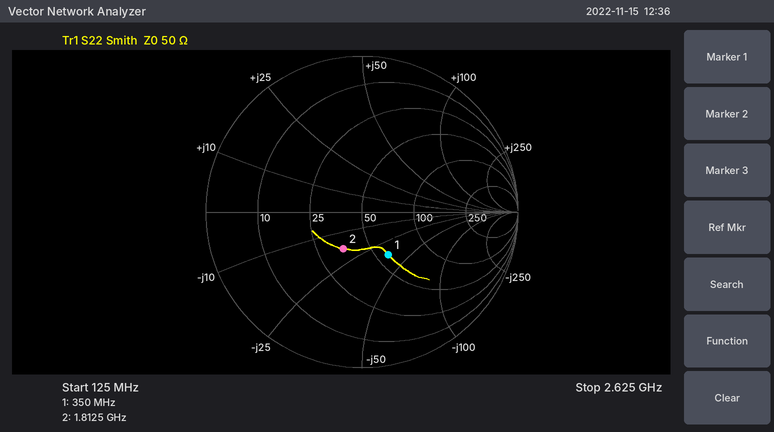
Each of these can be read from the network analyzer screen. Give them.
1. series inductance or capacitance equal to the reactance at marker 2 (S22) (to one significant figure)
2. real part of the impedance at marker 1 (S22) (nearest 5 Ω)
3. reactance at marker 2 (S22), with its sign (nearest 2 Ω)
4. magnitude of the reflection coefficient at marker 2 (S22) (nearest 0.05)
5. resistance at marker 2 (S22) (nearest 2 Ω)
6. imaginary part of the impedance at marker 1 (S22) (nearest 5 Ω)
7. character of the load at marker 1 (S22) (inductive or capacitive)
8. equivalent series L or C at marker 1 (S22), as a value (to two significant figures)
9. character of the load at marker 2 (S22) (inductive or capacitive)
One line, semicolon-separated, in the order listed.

5 pF; 60 Ω; -18 Ω; 0.25; 36 Ω; -35 Ω; capacitive; 13 pF; capacitive
